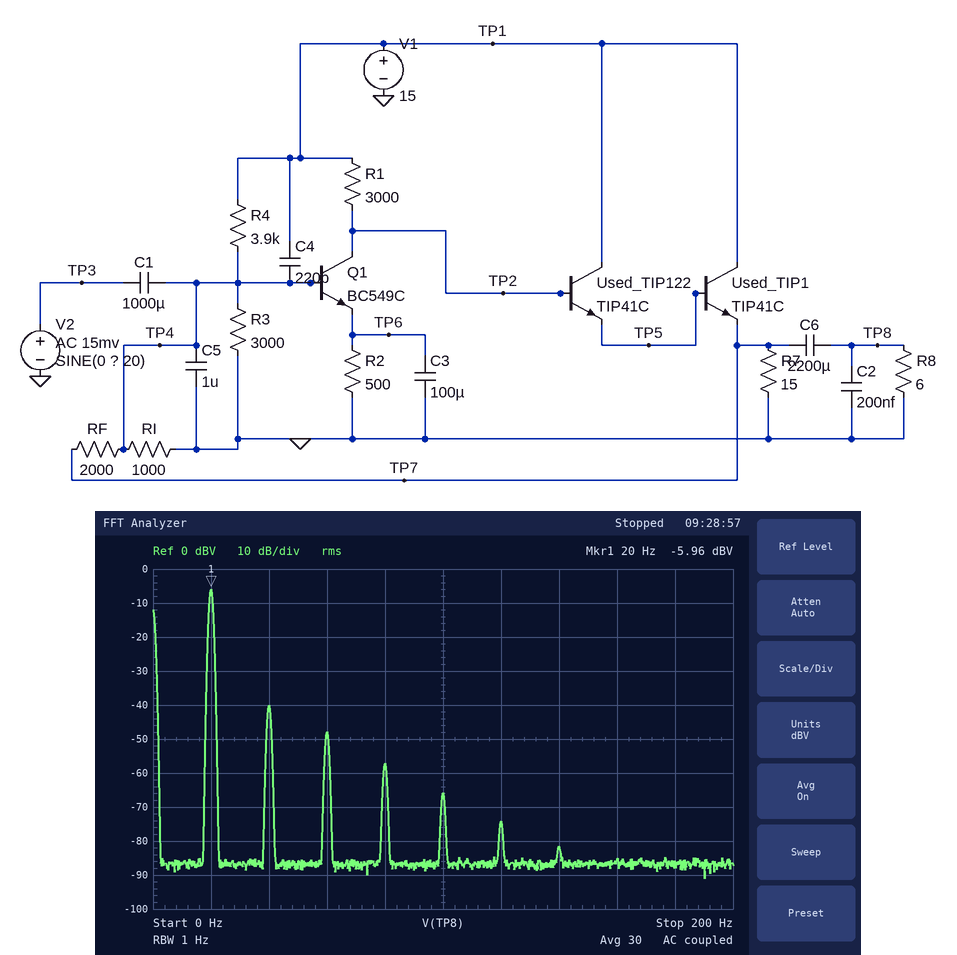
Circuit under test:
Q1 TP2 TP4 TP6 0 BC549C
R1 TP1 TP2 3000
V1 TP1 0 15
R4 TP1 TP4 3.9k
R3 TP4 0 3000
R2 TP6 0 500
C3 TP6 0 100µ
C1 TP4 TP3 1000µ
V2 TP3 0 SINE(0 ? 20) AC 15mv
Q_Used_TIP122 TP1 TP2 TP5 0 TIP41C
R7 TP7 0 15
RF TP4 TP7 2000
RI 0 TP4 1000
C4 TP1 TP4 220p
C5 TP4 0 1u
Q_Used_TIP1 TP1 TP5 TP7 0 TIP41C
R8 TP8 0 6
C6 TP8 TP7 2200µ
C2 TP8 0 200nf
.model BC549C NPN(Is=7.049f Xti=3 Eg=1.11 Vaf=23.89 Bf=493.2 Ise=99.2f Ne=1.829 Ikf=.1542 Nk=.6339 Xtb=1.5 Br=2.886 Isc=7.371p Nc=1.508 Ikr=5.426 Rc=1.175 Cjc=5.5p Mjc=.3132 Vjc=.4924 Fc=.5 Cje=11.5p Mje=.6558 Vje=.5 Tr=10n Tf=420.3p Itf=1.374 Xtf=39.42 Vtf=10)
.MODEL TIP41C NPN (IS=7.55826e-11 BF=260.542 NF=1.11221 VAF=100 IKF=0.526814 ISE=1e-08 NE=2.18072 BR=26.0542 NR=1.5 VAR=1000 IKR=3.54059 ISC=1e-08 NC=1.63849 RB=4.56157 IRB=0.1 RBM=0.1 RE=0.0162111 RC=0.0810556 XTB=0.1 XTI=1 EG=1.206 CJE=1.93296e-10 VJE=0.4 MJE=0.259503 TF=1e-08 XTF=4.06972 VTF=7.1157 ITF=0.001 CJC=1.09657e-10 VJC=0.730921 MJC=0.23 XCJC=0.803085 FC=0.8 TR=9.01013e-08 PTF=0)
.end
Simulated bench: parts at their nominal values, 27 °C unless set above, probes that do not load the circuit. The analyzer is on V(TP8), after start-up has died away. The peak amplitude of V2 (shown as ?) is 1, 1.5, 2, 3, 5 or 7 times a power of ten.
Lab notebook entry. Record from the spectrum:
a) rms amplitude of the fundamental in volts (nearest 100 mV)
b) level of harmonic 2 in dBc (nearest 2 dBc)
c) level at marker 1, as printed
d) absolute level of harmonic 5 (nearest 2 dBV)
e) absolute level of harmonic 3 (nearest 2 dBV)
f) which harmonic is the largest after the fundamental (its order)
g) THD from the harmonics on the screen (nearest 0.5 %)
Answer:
500 mV
-34 dBc
-5.96 dBV
-66 dBV
-48 dBV
2
2.0 %
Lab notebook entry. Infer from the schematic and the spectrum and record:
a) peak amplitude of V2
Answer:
30 mV
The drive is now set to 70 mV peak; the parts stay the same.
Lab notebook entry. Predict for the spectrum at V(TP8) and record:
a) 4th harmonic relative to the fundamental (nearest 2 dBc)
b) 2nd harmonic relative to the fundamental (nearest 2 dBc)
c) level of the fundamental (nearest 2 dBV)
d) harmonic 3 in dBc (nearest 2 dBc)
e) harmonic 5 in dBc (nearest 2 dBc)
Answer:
-32 dBc
-12 dBc
-2 dBV
-22 dBc
-30 dBc
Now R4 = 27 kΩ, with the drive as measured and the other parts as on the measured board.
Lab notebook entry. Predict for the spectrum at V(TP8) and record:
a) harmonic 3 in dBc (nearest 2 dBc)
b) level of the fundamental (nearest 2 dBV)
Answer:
-60 dBc
-6 dBV
